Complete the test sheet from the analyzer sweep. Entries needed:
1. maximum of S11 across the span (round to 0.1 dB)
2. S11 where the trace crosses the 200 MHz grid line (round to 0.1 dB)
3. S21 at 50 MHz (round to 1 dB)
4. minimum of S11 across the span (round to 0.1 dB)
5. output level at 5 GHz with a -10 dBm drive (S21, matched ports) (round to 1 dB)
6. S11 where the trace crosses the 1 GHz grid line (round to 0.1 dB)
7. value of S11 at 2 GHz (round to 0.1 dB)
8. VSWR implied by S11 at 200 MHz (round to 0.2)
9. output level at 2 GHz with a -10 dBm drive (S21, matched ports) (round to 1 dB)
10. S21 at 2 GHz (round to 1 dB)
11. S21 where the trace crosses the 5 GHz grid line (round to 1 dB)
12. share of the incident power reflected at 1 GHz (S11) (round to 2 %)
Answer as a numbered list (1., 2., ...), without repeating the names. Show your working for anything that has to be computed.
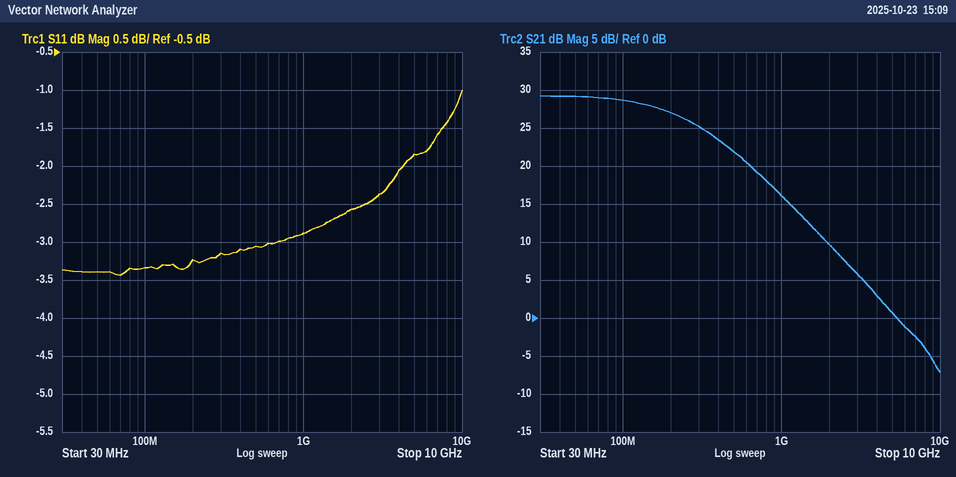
1. -1.0 dB
2. -3.2 dB
3. 29 dB
4. -3.4 dB
5. -10 dBm + (1 dB) = -9 dBm
6. -2.9 dB
7. -2.6 dB
8. |Γ| = 10^(-3.2/20) = 0.6918; VSWR = (1 + 0.6918)/(1 − 0.6918) ≈ 5.49, so 5.4 to the nearest 0.2
9. -10 dBm + (10 dB) = 0 dBm
10. 10 dB
11. 1 dB
12. 10^(-2.9/10) ≈ 51.3 %, so 52 % to the nearest 2 %
